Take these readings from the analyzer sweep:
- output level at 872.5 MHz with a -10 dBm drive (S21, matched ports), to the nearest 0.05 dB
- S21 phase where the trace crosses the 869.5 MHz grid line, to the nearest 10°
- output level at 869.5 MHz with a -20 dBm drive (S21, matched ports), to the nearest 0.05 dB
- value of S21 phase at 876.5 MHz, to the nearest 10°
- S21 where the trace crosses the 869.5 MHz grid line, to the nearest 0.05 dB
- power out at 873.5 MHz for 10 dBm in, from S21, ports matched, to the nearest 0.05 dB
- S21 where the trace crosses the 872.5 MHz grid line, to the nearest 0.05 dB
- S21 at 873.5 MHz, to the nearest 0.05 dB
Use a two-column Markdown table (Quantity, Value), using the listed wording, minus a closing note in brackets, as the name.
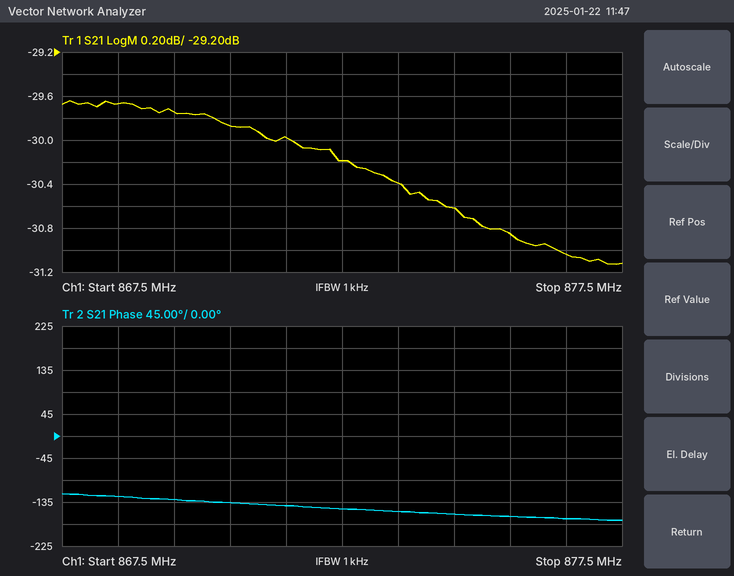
| Quantity | Value |
|---|---|
| output level at 872.5 MHz with a -10 dBm drive (S21, matched ports), to the nearest 0.05 dB | -40.20 dBm |
| S21 phase where the trace crosses the 869.5 MHz grid line, to the nearest 10° | -130° |
| output level at 869.5 MHz with a -20 dBm drive (S21, matched ports), to the nearest 0.05 dB | -49.75 dBm |
| value of S21 phase at 876.5 MHz, to the nearest 10° | -170° |
| S21 where the trace crosses the 869.5 MHz grid line, to the nearest 0.05 dB | -29.75 dB |
| power out at 873.5 MHz for 10 dBm in, from S21, ports matched, to the nearest 0.05 dB | -20.40 dBm |
| S21 where the trace crosses the 872.5 MHz grid line, to the nearest 0.05 dB | -30.20 dB |
| S21 at 873.5 MHz, to the nearest 0.05 dB | -30.40 dB |
